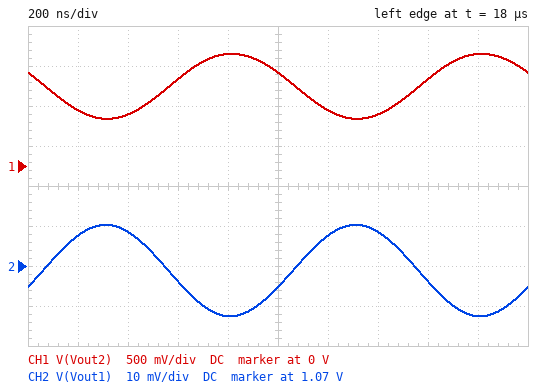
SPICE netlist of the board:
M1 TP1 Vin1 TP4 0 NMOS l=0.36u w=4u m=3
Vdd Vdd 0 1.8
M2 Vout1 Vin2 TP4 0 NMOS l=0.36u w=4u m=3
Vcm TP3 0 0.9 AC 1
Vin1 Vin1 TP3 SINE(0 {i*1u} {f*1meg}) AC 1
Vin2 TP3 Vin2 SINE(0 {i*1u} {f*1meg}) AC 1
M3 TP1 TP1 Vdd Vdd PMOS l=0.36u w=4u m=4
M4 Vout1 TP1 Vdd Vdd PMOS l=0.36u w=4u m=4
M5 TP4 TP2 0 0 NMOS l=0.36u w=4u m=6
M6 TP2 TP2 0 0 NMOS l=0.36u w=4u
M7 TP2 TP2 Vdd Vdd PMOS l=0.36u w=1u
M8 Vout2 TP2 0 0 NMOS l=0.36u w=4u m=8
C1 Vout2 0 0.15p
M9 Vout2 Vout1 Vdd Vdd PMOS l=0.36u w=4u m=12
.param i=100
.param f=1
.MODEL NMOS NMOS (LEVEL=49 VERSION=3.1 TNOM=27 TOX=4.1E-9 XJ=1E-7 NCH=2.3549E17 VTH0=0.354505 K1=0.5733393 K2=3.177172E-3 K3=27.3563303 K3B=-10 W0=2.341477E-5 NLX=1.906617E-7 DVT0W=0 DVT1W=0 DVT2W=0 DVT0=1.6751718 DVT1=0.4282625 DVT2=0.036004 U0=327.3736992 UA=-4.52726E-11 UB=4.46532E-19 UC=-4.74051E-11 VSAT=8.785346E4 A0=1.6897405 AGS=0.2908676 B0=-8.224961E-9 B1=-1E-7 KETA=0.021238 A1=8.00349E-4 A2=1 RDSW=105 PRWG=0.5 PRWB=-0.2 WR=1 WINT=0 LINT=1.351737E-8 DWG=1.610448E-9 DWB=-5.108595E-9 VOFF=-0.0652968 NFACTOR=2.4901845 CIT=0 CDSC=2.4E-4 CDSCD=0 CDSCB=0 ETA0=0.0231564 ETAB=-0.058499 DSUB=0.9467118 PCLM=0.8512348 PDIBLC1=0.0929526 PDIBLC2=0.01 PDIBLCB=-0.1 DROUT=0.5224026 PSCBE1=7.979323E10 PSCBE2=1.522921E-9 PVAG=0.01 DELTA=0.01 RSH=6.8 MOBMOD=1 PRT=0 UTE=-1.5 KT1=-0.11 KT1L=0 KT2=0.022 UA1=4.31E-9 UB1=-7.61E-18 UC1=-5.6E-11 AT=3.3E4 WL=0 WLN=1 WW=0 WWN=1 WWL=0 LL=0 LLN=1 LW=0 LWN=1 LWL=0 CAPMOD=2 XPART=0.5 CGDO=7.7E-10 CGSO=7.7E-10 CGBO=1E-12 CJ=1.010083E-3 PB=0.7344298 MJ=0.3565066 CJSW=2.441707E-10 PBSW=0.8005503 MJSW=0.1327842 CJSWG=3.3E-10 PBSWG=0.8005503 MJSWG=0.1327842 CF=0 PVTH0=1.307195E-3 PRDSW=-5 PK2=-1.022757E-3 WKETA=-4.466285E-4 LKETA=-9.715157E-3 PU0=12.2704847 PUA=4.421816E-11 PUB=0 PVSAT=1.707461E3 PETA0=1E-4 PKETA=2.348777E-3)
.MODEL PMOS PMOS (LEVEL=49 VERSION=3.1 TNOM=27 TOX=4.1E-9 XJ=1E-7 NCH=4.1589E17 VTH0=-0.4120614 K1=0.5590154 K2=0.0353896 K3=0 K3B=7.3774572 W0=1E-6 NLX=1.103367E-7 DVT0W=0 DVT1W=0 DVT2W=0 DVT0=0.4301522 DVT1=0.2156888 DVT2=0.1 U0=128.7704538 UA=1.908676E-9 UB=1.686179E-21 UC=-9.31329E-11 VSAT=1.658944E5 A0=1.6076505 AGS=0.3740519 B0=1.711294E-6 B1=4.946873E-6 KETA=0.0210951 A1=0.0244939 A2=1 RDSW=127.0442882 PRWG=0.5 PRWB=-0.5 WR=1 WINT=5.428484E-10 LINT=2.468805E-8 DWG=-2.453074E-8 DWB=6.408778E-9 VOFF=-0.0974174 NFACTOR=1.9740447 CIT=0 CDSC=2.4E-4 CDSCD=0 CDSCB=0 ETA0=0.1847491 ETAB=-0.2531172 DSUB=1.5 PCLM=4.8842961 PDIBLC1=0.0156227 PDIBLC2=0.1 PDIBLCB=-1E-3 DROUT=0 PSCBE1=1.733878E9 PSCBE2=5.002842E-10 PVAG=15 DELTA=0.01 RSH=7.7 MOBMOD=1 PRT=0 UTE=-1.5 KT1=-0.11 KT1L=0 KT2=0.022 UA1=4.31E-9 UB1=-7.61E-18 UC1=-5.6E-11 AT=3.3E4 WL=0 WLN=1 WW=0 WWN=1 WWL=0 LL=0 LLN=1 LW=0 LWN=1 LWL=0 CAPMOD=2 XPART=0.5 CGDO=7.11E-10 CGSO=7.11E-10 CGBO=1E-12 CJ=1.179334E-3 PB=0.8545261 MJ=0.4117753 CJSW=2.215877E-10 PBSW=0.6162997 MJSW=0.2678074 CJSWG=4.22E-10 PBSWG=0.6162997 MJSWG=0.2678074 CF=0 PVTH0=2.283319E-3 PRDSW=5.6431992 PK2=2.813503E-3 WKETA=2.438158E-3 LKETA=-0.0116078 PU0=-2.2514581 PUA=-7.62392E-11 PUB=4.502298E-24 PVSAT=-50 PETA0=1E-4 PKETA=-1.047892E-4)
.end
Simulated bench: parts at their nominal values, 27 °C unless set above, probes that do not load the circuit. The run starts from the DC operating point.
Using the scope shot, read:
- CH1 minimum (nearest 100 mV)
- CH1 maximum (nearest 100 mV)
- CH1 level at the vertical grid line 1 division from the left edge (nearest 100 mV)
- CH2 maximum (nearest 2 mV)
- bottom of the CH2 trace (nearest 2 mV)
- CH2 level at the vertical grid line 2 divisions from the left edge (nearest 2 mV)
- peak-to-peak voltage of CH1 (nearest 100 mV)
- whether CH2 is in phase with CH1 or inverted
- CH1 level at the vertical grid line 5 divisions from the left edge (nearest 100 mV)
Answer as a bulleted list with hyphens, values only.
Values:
- 600 mV
- 1.4 V
- 700 mV
- 1.080 V
- 1.058 V
- 1.078 V
- 800 mV
- inverted
- 1.2 V
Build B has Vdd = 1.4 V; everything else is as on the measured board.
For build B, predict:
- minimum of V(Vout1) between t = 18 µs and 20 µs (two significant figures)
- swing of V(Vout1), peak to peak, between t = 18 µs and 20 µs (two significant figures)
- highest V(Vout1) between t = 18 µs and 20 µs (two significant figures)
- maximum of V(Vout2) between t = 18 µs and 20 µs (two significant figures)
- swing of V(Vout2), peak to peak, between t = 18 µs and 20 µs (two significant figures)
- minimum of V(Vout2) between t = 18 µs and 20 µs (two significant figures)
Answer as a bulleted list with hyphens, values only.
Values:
- 780 mV
- 18 mV
- 800 mV
- 1.2 V
- 760 mV
- 470 mV
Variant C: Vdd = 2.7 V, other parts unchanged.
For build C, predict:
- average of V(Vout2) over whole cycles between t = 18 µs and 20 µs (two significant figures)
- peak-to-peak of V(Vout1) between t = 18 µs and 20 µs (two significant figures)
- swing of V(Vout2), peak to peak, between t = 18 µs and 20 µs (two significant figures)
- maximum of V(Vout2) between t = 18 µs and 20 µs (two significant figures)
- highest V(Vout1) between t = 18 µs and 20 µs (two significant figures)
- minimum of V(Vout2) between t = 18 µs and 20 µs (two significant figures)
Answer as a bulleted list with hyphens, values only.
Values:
- 210 mV
- 19 mV
- 45 mV
- 240 mV
- 1.8 V
- 190 mV
